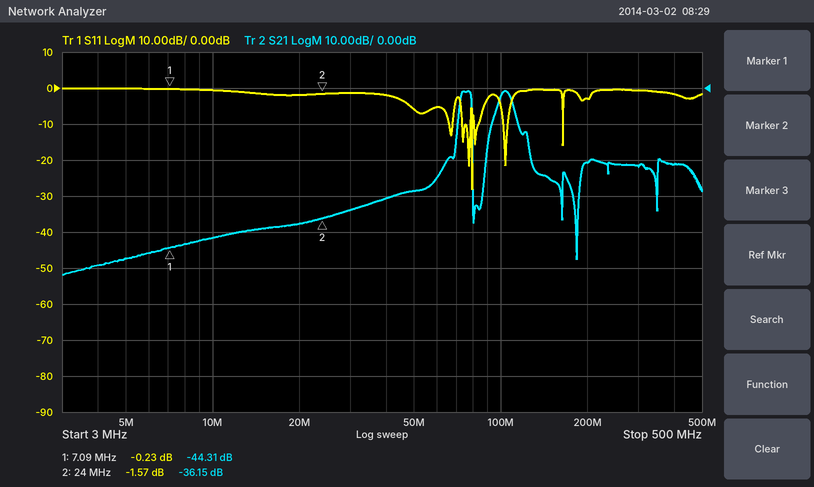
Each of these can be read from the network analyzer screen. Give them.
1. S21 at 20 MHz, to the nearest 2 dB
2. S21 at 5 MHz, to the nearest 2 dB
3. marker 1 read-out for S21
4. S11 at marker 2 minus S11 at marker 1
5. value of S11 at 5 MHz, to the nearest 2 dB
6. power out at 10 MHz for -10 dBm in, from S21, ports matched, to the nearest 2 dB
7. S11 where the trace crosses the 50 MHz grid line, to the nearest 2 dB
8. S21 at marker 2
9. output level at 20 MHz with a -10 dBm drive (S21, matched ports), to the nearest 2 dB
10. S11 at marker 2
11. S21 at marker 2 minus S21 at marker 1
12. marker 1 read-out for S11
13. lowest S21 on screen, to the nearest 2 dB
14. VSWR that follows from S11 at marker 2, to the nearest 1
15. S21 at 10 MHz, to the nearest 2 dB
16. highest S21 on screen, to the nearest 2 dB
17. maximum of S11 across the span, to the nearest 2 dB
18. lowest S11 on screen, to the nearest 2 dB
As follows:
-38 dB
-48 dB
-44.31 dB
-1.34 dB
0 dB
-52 dBm
-6 dB
-36.15 dB
-48 dBm
-1.57 dB
8.16 dB
-0.23 dB
-52 dB
11
-42 dB
0 dB
0 dB
-28 dB
